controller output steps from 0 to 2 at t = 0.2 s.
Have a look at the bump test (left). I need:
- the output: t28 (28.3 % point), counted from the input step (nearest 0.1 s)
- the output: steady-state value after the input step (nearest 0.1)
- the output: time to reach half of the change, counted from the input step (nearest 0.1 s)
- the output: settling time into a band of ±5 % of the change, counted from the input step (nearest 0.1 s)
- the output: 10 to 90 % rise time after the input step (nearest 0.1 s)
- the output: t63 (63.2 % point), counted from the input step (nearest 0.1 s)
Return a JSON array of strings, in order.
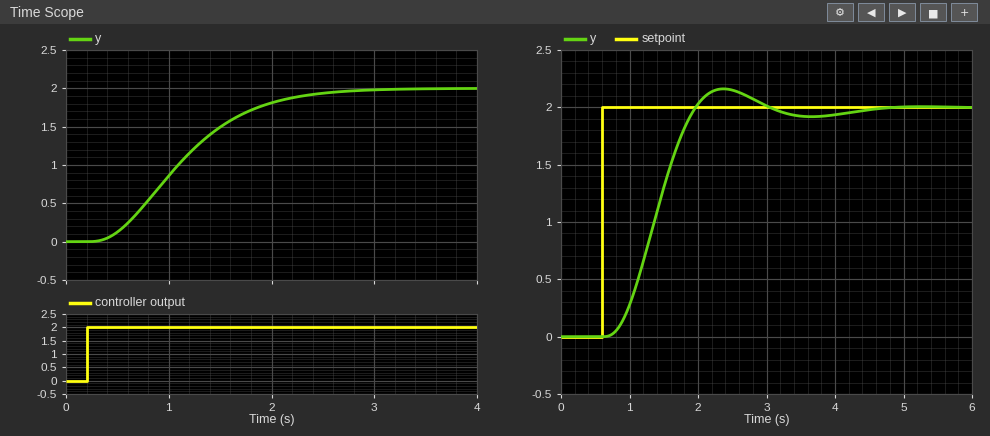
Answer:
["0.6 s", "2.0", "0.9 s", "2.1 s", "1.4 s", "1.1 s"]
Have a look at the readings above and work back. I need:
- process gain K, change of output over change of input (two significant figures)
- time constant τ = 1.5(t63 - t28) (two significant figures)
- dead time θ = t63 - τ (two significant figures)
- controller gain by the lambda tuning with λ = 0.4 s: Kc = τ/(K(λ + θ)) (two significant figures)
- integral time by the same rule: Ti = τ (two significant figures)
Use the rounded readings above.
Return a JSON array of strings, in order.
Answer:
["1.0", "0.75 s", "0.35 s", "1.0", "0.75 s"]
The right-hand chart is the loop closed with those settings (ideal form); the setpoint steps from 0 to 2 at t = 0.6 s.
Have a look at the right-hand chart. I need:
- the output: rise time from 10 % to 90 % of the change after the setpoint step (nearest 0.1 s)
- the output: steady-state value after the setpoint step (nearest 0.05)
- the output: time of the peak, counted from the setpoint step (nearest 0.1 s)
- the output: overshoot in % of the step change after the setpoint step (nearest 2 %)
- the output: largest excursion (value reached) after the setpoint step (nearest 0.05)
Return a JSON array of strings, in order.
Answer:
["0.8 s", "2.00", "1.8 s", "8 %", "2.15"]
